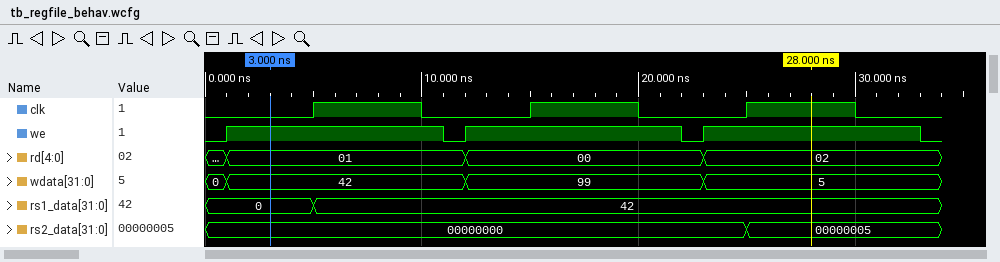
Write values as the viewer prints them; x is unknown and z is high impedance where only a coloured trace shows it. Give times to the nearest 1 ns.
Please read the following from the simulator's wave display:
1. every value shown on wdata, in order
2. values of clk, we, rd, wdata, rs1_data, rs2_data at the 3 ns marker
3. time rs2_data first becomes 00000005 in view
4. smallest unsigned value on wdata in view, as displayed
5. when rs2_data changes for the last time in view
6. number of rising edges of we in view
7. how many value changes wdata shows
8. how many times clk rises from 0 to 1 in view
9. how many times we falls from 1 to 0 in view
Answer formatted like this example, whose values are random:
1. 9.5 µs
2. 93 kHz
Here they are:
1. 0, 42, 99, 5
2. clk=0, we=1, rd=01, wdata=42, rs1_data=0, rs2_data=00000000
3. 25 ns
4. 0
5. 25 ns
6. 3
7. 3
8. 3
9. 3
